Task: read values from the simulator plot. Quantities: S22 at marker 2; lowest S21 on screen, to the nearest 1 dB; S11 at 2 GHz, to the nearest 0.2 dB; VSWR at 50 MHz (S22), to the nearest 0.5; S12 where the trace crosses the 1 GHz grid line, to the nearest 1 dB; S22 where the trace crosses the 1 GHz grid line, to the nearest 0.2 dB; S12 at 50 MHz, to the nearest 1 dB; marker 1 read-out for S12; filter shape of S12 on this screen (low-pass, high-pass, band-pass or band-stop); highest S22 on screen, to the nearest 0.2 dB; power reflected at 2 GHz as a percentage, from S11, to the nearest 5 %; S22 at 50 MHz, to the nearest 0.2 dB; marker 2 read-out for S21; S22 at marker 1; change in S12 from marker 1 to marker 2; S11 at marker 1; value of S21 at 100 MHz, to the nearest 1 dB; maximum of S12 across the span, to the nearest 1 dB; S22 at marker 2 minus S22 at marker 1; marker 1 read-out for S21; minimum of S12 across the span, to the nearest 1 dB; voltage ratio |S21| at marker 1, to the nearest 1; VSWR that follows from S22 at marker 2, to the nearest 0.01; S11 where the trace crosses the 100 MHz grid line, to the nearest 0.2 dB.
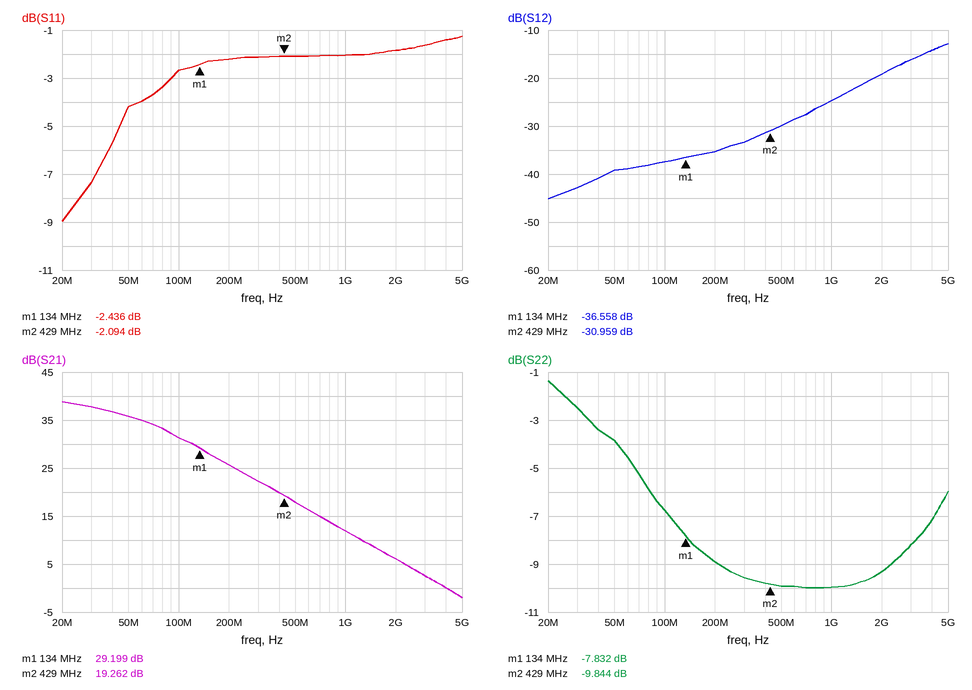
-9.844 dB
-2 dB
-1.8 dB
4.5
-25 dB
-10.0 dB
-39 dB
-36.558 dB
high-pass
-1.4 dB
65 %
-3.8 dB
19.262 dB
-7.832 dB
5.599 dB
-2.436 dB
31 dB
-13 dB
-2.012 dB
29.199 dB
-45 dB
29
1.95
-2.6 dB
